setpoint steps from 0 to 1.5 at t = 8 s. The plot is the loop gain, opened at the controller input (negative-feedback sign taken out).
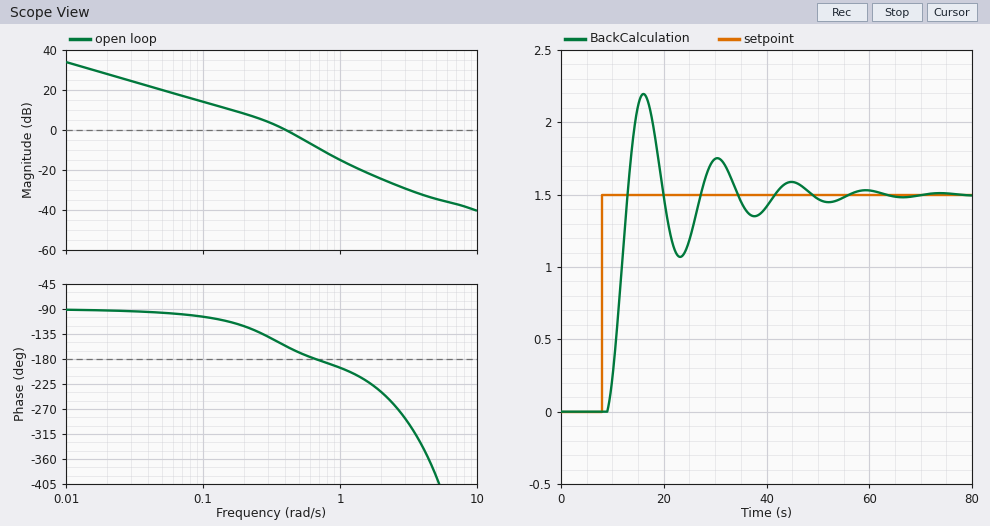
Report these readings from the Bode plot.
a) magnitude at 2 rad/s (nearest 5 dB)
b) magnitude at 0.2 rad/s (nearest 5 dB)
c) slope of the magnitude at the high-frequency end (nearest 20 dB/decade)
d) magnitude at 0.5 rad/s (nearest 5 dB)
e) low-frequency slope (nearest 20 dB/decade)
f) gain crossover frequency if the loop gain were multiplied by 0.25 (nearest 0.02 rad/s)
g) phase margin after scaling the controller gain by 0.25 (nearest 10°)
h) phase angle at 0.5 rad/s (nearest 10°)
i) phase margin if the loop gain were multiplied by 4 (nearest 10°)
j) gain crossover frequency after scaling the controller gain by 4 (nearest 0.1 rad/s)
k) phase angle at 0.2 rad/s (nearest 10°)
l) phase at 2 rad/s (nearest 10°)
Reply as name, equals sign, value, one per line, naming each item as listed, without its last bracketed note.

magnitude at 2 rad/s = -25 dB
magnitude at 0.2 rad/s = 10 dB
slope of the magnitude at the high-frequency end = -20 dB/decade
magnitude at 0.5 rad/s = -5 dB
low-frequency slope = -20 dB/decade
gain crossover frequency if the loop gain were multiplied by 0.25 = 0.12 rad/s
phase margin after scaling the controller gain by 0.25 = 70°
phase angle at 0.5 rad/s = -170°
phase margin if the loop gain were multiplied by 4 = -10°
gain crossover frequency after scaling the controller gain by 4 = 0.8 rad/s
phase angle at 0.2 rad/s = -120°
phase at 2 rad/s = -240°
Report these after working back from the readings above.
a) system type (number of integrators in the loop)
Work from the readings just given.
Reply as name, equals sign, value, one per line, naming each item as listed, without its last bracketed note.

system type = 1
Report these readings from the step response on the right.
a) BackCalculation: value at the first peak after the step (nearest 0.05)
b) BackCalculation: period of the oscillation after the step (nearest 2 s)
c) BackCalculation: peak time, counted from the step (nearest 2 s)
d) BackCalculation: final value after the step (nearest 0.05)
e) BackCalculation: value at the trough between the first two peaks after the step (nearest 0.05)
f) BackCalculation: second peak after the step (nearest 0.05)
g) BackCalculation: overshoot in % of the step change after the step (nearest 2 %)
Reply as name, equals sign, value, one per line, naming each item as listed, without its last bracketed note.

BackCalculation: value at the first peak after the step = 2.20
BackCalculation: period of the oscillation after the step = 14 s
BackCalculation: peak time, counted from the step = 8 s
BackCalculation: final value after the step = 1.50
BackCalculation: value at the trough between the first two peaks after the step = 1.05
BackCalculation: second peak after the step = 1.75
BackCalculation: overshoot in % of the step change after the step = 46 %
